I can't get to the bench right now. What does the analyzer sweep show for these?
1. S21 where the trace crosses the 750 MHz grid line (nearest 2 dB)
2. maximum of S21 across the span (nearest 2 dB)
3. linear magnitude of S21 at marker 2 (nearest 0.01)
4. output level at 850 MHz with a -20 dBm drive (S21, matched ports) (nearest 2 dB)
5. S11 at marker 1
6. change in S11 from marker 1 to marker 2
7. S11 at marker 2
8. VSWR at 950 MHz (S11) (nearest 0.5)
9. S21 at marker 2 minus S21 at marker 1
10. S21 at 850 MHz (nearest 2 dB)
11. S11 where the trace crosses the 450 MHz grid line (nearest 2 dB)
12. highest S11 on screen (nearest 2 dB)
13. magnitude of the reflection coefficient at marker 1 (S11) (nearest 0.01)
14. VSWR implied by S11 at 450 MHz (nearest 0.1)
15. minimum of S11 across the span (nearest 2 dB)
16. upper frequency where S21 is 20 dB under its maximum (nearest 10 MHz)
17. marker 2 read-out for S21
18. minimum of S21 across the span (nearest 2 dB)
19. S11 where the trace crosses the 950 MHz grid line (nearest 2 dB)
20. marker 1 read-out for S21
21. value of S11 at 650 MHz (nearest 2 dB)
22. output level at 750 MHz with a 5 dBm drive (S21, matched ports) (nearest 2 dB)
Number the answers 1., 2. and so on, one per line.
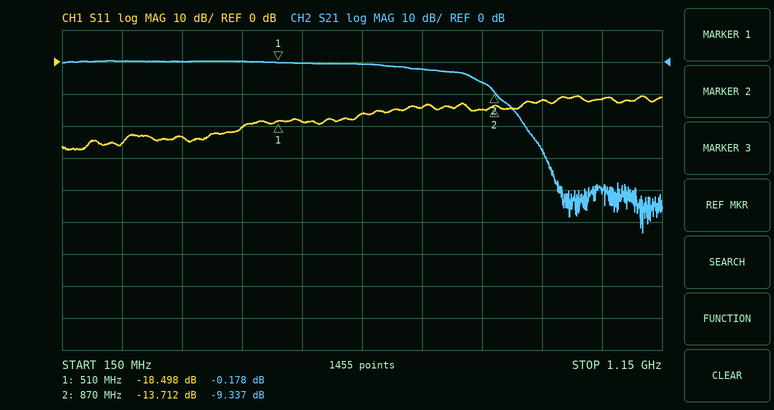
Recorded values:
1. -2 dB
2. 0 dB
3. 0.34
4. -26 dBm
5. -18.498 dB
6. 4.786 dB
7. -13.712 dB
8. 1.5
9. -9.159 dB
10. -6 dB
11. -20 dB
12. -10 dB
13. 0.12
14. 1.2
15. -28 dB
16. 920 MHz
17. -9.337 dB
18. -54 dB
19. -12 dB
20. -0.178 dB
21. -16 dB
22. 2 dBm
